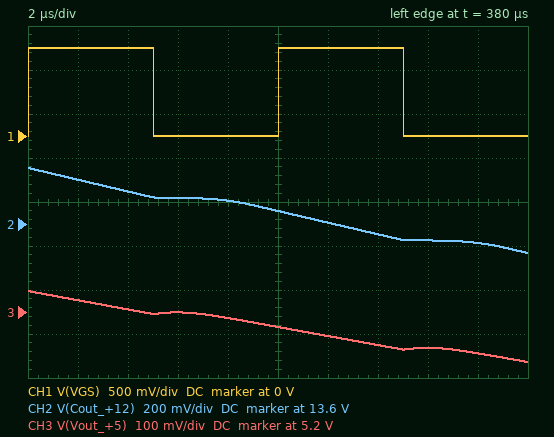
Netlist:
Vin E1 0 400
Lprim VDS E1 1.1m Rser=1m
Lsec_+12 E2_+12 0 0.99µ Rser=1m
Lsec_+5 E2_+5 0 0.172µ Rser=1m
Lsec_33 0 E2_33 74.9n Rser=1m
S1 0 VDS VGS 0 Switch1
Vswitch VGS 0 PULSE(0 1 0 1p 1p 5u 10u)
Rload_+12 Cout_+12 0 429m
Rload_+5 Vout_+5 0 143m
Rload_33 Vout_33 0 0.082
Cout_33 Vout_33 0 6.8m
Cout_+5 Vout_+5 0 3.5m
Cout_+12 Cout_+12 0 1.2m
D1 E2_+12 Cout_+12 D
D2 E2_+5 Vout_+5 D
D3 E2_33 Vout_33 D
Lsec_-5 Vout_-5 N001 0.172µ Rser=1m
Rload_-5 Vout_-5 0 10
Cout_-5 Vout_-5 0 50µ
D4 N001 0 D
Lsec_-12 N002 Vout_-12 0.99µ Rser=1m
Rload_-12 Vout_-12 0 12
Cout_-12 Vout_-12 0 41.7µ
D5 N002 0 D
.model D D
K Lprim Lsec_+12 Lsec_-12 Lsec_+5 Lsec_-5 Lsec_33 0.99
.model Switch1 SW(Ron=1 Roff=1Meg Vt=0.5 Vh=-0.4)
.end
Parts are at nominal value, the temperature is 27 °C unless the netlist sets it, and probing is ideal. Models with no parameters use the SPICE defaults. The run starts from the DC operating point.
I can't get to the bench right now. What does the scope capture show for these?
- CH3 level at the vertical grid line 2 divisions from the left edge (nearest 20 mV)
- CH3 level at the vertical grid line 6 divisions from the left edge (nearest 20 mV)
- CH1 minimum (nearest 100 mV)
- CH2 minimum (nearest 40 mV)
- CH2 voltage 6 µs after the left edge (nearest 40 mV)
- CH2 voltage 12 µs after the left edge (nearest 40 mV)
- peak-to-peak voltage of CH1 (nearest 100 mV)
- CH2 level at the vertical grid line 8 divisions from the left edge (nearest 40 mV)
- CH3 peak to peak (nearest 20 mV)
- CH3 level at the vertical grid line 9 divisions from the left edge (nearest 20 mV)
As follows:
5.20 V
5.14 V
0 V
13.48 V
13.72 V
13.60 V
1.0 V
13.52 V
160 mV
5.10 V
